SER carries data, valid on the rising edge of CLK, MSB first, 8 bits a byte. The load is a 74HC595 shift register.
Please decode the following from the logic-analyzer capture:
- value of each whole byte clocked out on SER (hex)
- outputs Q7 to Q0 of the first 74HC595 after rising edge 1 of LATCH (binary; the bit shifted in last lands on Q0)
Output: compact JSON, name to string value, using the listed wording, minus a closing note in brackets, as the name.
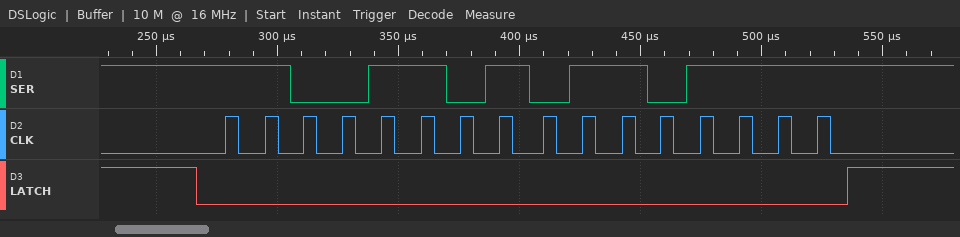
{"value of each whole byte clocked out on SER": "0xCD 0x6F", "outputs Q7 to Q0 of the first 74HC595 after rising edge 1 of LATCH": "01101111"}
